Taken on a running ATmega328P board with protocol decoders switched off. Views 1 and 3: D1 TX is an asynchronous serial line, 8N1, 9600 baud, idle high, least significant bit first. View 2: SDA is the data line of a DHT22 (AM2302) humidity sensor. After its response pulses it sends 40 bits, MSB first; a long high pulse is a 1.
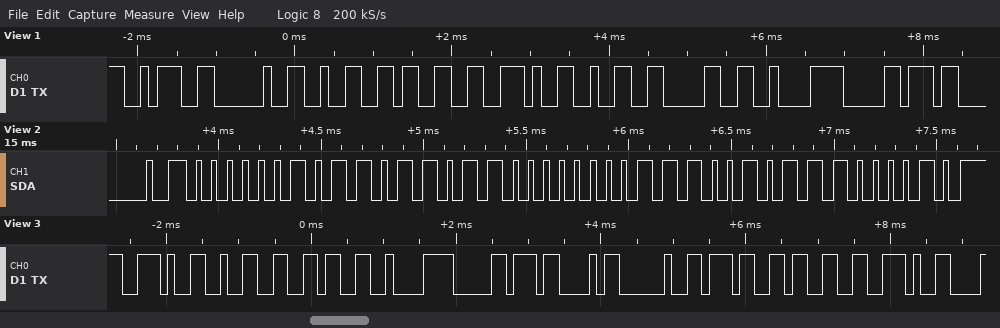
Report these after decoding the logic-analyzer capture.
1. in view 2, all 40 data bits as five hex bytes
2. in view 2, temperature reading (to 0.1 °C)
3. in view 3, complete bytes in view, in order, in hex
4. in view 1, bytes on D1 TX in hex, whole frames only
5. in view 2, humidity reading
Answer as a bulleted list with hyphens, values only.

- 02 DB 00 E5 C2
- 22.9 °C
- 2E 32 36 C2 B0 43 20 37 33 2E
- 3A 20 32 33 2E 32 30 C2 B0
- 73.1 %
